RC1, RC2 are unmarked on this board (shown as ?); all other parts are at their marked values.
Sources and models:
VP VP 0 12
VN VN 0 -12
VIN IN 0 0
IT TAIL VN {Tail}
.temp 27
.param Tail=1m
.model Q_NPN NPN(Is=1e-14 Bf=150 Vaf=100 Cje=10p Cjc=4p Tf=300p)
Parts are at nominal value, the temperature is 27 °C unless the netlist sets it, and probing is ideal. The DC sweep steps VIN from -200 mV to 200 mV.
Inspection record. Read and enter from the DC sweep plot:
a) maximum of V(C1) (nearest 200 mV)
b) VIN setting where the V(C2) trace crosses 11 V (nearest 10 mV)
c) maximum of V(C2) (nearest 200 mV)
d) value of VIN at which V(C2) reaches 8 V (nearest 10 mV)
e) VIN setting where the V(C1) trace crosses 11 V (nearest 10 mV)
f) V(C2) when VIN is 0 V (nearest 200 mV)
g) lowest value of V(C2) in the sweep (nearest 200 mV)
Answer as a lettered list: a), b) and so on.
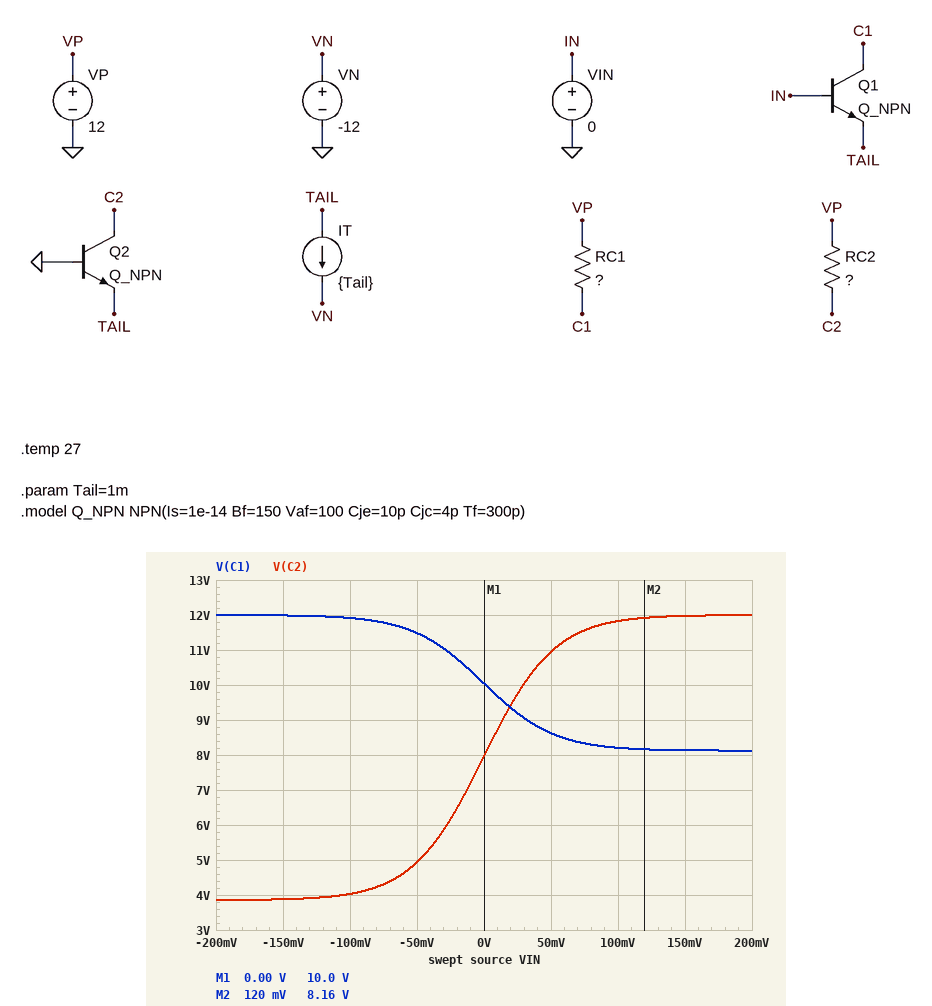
a) 12.0 V
b) 50 mV
c) 12.0 V
d) 0 V
e) -30 mV
f) 8.0 V
g) 3.8 V
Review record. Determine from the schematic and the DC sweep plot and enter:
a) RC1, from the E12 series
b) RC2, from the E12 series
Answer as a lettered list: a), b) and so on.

a) 3.9 kΩ
b) 8.2 kΩ
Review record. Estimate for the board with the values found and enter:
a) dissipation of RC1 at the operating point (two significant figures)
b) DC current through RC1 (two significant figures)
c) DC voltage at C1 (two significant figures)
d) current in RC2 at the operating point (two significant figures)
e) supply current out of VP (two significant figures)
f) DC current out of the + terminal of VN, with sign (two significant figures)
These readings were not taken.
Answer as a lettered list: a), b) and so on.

a) 980 µW
b) 500 µA
c) 10 V
d) 490 µA
e) 990 µA
f) -1.0 mA
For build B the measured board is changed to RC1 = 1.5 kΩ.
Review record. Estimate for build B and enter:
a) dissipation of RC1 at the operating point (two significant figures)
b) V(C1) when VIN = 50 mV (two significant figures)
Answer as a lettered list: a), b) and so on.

a) 380 µW
b) 11 V
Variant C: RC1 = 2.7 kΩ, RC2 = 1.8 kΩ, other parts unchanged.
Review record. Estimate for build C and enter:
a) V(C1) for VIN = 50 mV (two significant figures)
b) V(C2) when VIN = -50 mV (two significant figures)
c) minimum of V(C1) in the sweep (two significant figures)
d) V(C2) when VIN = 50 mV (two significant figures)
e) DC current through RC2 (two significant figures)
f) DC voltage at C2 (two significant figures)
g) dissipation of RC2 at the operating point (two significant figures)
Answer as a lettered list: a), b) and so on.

a) 9.7 V
b) 10 V
c) 9.3 V
d) 12 V
e) 500 µA
f) 11 V
g) 450 µW
